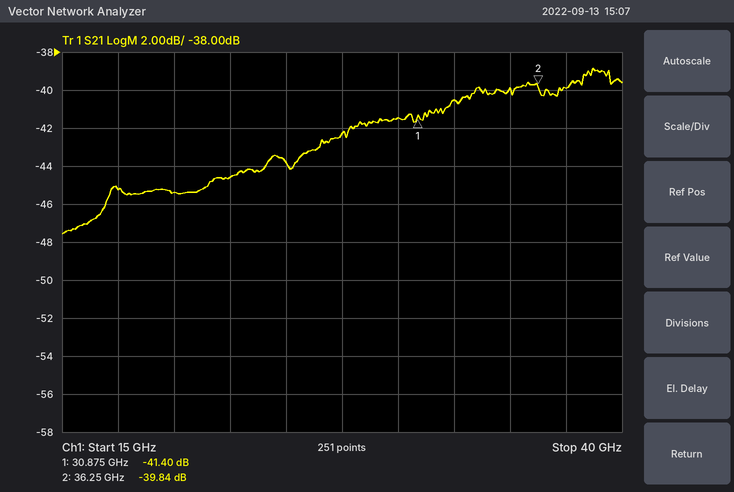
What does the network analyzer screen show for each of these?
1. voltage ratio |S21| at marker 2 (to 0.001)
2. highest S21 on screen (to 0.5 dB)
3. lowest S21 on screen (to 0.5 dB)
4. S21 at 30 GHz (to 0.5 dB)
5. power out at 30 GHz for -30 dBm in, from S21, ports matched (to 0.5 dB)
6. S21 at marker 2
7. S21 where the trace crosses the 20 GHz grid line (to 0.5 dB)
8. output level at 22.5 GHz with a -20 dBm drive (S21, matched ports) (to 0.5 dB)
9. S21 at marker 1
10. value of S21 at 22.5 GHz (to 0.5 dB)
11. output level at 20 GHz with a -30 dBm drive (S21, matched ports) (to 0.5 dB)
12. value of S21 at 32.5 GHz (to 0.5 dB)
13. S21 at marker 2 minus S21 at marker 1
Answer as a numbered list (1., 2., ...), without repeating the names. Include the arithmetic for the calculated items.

1. 10^(-39.84/20) ≈ 0.010
2. -39.0 dB
3. -47.5 dB
4. -41.5 dB
5. -30 dBm + (-41.5 dB) = -71.5 dBm
6. -39.84 dB
7. -45.5 dB
8. -20 dBm + (-44.5 dB) = -64.5 dBm
9. -41.40 dB
10. -44.5 dB
11. -30 dBm + (-45.5 dB) = -75.5 dBm
12. -40.5 dB
13. -39.84 − (-41.4) = 1.56 dB
